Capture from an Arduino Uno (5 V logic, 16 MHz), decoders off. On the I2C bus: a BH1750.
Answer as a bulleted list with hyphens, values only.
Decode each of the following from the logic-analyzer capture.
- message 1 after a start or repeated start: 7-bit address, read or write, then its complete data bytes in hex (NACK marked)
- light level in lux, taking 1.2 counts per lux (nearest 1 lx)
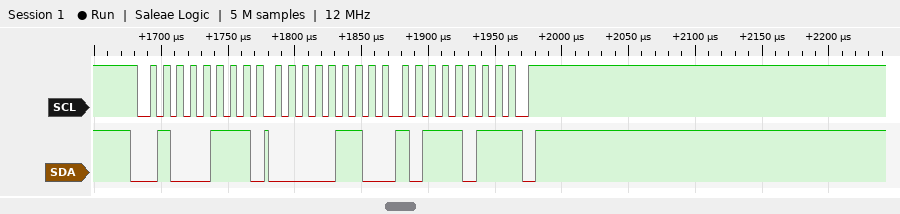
- 0x23 read: 06 BB NACK
- 1436 lx
